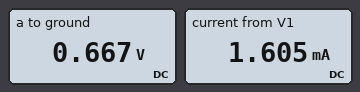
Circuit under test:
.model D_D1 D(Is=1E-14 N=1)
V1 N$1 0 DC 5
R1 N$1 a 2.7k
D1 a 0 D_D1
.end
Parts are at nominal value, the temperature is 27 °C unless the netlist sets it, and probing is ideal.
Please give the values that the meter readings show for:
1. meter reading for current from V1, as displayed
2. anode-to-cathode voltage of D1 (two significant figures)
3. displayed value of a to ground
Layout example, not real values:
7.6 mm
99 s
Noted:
1.605 mA
670 mV
0.667 V
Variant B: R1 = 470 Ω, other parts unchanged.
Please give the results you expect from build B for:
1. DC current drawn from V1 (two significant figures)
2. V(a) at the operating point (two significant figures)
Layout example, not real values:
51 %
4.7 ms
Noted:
9.1 mA
710 mV
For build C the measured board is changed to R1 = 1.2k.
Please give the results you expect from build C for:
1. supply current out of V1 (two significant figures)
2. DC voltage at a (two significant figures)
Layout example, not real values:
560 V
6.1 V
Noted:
3.6 mA
690 mV
